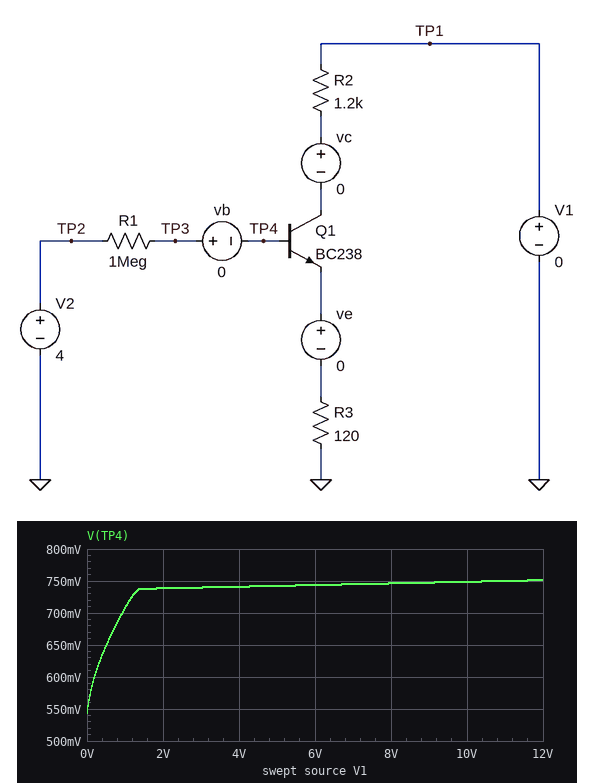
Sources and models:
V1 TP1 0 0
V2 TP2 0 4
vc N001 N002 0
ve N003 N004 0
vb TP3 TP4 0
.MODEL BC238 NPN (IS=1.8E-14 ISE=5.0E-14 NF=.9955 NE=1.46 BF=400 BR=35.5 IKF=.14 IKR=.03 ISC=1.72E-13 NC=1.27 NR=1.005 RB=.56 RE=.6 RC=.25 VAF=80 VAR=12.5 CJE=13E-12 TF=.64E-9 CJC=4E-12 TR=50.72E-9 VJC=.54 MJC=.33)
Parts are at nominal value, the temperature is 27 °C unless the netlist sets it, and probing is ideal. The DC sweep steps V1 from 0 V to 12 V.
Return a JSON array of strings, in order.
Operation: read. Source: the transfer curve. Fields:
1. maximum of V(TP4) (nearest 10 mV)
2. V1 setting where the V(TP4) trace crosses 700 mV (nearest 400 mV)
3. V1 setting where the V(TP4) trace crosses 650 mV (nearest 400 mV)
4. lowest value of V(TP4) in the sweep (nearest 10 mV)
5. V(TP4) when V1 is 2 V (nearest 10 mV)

["750 mV", "800 mV", "400 mV", "540 mV", "740 mV"]
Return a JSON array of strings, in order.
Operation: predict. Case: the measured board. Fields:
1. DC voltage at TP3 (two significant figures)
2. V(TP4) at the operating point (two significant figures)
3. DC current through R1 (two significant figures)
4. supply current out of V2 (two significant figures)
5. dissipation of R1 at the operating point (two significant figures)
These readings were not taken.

["540 mV", "540 mV", "3.5 µA", "3.5 µA", "12 µW"]
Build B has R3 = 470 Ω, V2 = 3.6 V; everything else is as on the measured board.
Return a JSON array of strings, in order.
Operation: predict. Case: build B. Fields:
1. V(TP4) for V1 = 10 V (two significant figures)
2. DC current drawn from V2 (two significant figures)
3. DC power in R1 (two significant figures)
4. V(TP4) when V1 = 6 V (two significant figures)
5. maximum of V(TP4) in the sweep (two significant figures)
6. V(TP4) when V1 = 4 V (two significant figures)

["980 mV", "3.1 µA", "9.4 µW", "970 mV", "990 mV", "960 mV"]
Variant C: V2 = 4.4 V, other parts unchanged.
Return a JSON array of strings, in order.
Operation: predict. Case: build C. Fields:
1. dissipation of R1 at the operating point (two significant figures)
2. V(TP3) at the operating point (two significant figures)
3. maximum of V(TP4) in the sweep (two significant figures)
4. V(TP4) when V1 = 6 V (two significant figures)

["15 µW", "550 mV", "770 mV", "760 mV"]
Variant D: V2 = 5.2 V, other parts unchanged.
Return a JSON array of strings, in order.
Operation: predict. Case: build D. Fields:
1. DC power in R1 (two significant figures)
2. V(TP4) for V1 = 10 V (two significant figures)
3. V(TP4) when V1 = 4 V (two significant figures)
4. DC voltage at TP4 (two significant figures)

["22 µW", "800 mV", "790 mV", "550 mV"]
